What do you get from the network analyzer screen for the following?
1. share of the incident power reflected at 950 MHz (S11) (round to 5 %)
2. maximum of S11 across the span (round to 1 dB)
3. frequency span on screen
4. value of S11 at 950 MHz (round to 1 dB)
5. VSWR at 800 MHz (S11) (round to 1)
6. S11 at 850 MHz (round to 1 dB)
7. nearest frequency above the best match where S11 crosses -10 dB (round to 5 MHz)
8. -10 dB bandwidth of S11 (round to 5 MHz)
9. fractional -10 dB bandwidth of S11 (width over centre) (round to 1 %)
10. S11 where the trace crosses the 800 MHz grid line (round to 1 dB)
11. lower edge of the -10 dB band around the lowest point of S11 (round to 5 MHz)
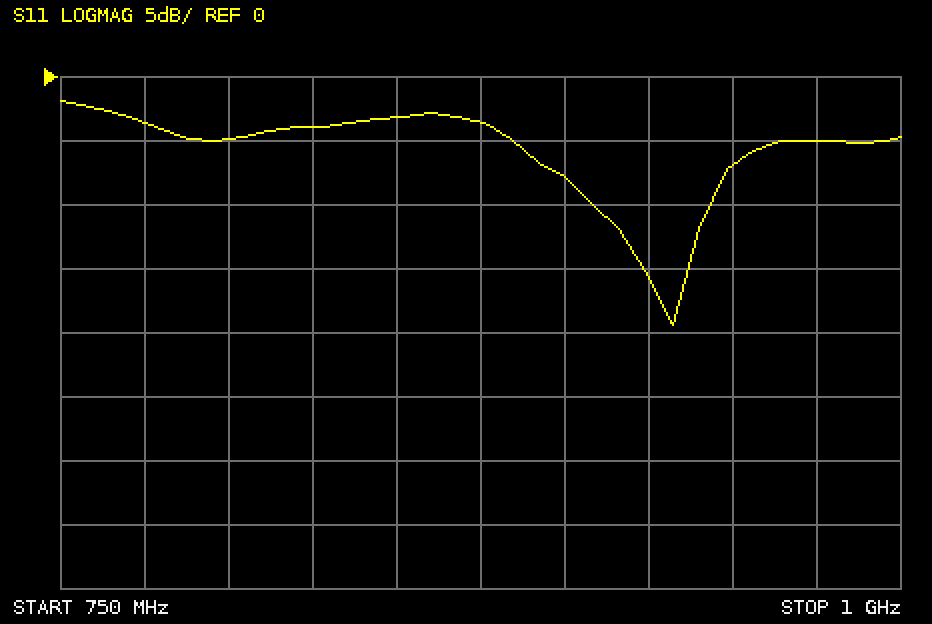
20 %
-2 dB
250 MHz
-7 dB
4
-3 dB
945 MHz
35 MHz
4 %
-5 dB
910 MHz
